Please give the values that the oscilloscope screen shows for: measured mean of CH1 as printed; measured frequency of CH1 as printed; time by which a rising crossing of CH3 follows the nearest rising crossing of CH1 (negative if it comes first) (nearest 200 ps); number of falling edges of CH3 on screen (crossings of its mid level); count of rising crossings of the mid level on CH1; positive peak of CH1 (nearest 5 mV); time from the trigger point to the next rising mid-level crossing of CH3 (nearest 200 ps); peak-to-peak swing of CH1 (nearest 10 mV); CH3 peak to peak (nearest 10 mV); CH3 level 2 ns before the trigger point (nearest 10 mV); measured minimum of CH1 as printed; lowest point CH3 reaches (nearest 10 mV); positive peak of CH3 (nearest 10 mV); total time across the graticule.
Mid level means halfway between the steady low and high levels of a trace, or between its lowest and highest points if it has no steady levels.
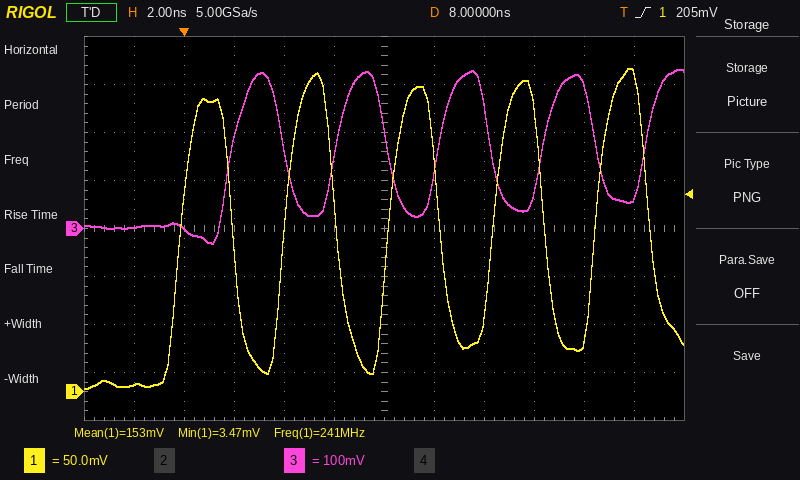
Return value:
153 mV
241 MHz
+2.0 ns
4
5
335 mV
1.8 ns
330 mV
360 mV
0 mV
3.47 mV
-30 mV
330 mV
24 ns
